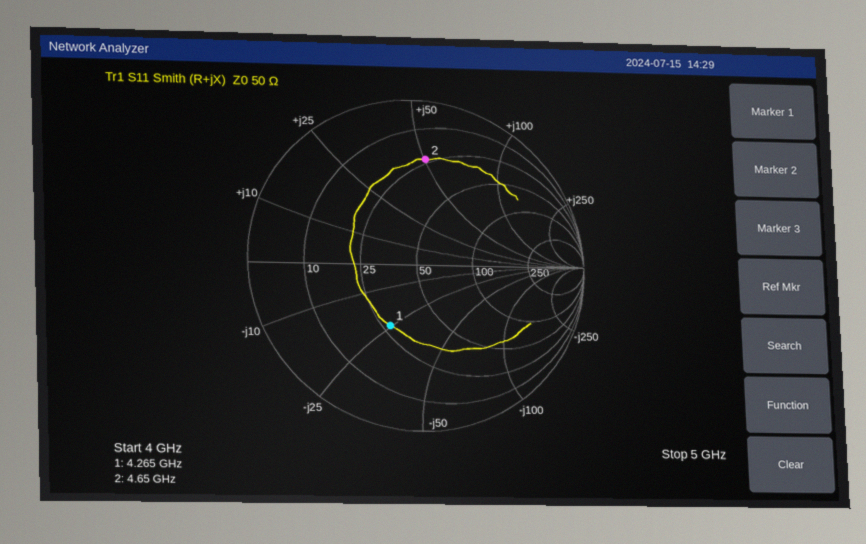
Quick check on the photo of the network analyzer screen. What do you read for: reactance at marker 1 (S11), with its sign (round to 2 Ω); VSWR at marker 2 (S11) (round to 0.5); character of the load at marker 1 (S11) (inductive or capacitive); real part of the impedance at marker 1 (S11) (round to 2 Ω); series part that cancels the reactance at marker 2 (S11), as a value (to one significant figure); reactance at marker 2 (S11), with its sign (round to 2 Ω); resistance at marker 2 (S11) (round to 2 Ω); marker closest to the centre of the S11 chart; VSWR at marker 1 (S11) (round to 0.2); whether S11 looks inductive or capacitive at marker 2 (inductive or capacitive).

-24 Ω
4.5
capacitive
28 Ω
700 fF
+50 Ω
24 Ω
marker 1
2.4
inductive
